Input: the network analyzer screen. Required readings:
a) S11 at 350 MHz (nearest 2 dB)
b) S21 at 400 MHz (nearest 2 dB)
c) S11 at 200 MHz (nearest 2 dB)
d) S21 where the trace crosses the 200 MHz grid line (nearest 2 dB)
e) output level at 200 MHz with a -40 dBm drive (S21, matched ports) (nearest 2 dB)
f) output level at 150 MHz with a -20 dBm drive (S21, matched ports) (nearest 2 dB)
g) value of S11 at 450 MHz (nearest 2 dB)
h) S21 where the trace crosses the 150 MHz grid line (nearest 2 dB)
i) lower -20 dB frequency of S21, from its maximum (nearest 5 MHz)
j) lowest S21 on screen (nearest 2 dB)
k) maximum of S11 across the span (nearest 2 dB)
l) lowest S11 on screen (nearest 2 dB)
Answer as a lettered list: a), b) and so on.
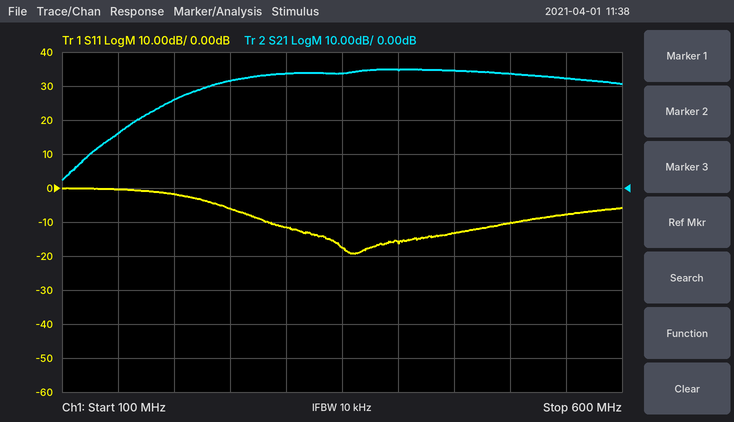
a) -18 dB
b) 34 dB
c) -2 dB
d) 26 dB
e) -14 dBm
f) -4 dBm
g) -14 dB
h) 16 dB
i) 145 MHz
j) 2 dB
k) 0 dB
l) -20 dB
